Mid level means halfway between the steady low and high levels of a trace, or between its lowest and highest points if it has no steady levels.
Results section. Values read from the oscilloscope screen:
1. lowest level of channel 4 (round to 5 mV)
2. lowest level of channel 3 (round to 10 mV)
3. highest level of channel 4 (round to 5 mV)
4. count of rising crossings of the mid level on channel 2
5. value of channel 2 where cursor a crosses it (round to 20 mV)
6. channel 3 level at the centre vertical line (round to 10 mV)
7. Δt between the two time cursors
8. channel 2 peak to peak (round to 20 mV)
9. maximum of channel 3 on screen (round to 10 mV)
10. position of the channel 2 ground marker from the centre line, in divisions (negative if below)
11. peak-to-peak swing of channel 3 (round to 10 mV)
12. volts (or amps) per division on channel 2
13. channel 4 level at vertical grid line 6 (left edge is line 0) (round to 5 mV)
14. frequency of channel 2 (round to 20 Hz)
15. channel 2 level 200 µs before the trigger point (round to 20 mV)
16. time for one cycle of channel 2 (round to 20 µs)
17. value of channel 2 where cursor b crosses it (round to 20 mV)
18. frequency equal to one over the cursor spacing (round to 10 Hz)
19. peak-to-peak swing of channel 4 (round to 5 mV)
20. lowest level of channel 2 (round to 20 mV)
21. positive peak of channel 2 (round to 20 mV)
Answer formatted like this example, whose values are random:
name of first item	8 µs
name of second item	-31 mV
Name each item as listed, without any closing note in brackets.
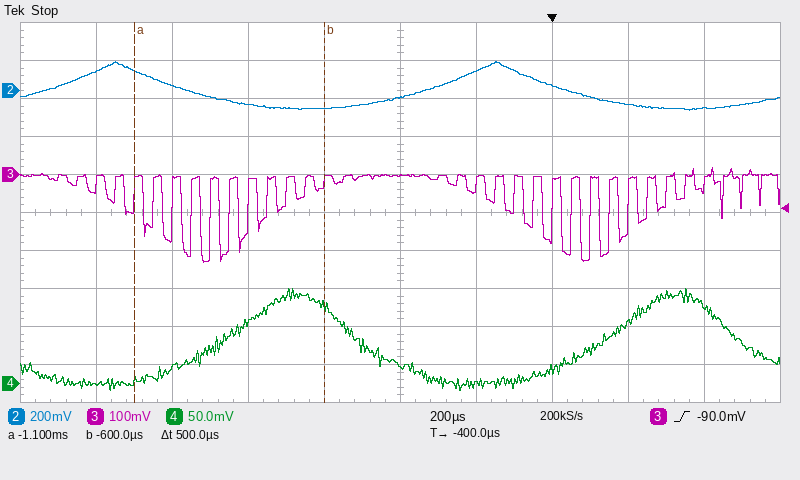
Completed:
lowest level of channel 4	-10 mV
lowest level of channel 3	-230 mV
highest level of channel 4	125 mV
count of rising crossings of the mid level on channel 2	2
value of channel 2 where cursor a crosses it	100 mV
channel 3 level at the centre vertical line	0 mV
Δt between the two time cursors	500 µs
channel 2 peak to peak	260 mV
maximum of channel 3 on screen	20 mV
position of the channel 2 ground marker from the centre line, in divisions	+3.2 div
peak-to-peak swing of channel 3	250 mV
volts (or amps) per division on channel 2	200 mV
channel 4 level at vertical grid line 6 (left edge is line 0)	0 mV
frequency of channel 2	1.00 kHz
channel 2 level 200 µs before the trigger point	100 mV
time for one cycle of channel 2	1.00 ms
value of channel 2 where cursor b crosses it	-100 mV
frequency equal to one over the cursor spacing	2.00 kHz
peak-to-peak swing of channel 4	135 mV
lowest level of channel 2	-100 mV
positive peak of channel 2	160 mV
